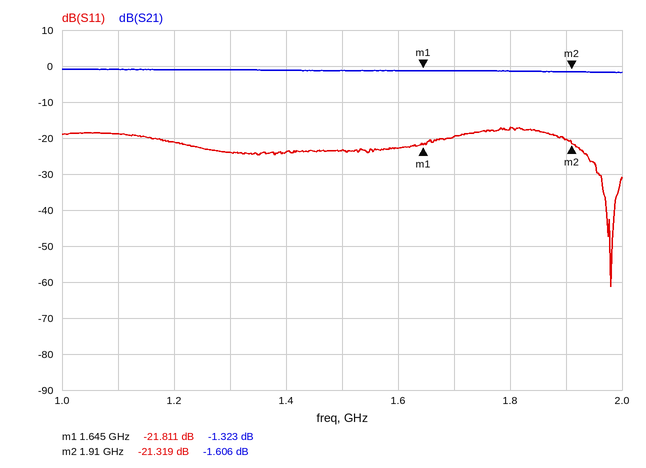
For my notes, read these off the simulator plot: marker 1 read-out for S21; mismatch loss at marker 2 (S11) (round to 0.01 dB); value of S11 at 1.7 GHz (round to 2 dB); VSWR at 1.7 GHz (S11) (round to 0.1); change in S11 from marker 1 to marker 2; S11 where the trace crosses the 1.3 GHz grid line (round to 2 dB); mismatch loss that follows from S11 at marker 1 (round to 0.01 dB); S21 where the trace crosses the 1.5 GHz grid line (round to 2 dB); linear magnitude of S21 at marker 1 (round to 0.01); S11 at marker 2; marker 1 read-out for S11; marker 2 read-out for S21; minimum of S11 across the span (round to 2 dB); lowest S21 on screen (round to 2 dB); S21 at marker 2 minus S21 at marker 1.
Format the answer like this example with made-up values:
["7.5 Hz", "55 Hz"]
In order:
["-1.323 dB", "0.03 dB", "-20 dB", "1.2", "0.492 dB", "-24 dB", "0.03 dB", "-2 dB", "0.86", "-21.319 dB", "-21.811 dB", "-1.606 dB", "-62 dB", "-2 dB", "-0.283 dB"]
